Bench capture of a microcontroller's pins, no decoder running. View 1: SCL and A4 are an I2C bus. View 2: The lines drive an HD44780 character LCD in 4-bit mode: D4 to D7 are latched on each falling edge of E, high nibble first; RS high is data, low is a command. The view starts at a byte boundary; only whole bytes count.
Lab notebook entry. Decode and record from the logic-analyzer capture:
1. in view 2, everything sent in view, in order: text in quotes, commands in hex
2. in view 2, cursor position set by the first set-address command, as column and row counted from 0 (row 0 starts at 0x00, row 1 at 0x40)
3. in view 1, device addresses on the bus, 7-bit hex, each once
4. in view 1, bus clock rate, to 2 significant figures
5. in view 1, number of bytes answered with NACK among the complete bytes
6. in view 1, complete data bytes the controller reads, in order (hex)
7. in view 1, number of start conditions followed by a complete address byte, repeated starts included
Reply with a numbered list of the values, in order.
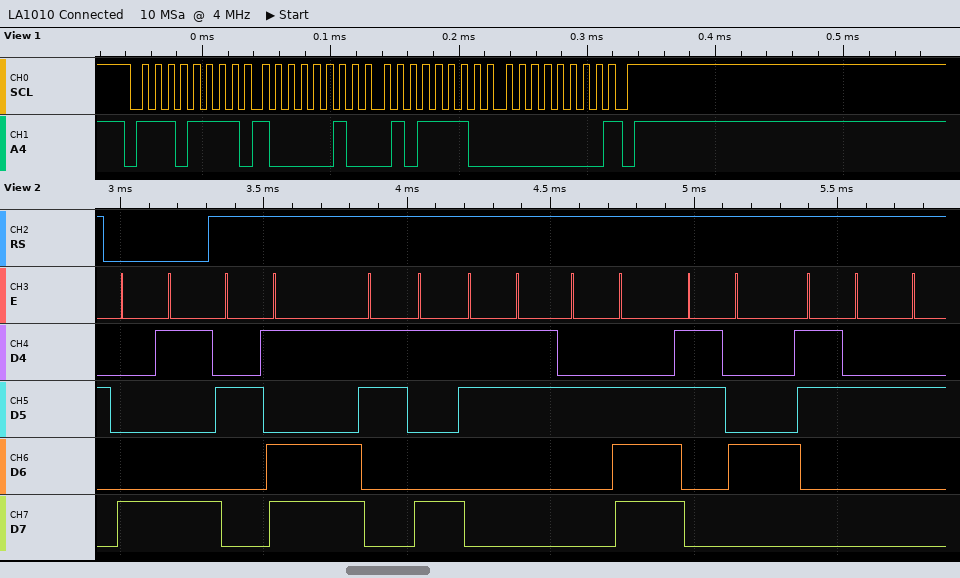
1. 0x89 "-93.42"
2. column 9, row 0
3. 0x77
4. 100 kHz
5. 1
6. 82 5E 00
7. 1
